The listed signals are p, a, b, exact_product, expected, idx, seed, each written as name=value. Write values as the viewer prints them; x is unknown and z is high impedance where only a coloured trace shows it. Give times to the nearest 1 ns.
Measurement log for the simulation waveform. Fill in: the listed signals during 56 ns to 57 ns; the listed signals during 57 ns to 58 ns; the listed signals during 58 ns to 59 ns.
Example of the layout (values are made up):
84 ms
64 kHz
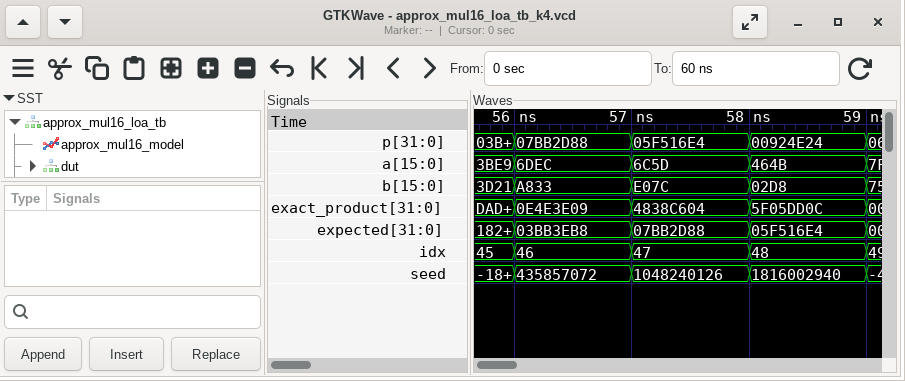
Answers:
p=07BB2D88, a=6DEC, b=A833, exact_product=0E4E3E09, expected=03BB3EB8, idx=46, seed=435857072
p=05F516E4, a=6C5D, b=E07C, exact_product=4838C604, expected=07BB2D88, idx=47, seed=1048240126
p=00924E24, a=464B, b=02D8, exact_product=5F05DD0C, expected=05F516E4, idx=48, seed=1816002940
